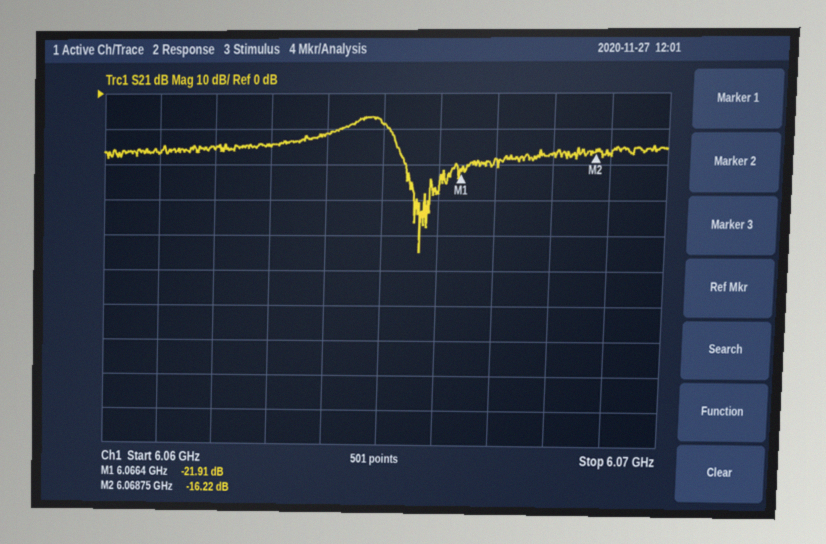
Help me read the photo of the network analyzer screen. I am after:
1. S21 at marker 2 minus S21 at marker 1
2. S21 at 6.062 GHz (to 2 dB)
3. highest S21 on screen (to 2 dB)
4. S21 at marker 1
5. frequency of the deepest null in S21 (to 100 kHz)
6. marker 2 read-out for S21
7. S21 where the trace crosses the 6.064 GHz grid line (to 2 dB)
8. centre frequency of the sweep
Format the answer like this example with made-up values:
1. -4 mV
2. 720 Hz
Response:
1. 5.69 dB
2. -16 dB
3. -6 dB
4. -21.91 dB
5. 6.0657 GHz
6. -16.22 dB
7. -12 dB
8. 6.065 GHz
